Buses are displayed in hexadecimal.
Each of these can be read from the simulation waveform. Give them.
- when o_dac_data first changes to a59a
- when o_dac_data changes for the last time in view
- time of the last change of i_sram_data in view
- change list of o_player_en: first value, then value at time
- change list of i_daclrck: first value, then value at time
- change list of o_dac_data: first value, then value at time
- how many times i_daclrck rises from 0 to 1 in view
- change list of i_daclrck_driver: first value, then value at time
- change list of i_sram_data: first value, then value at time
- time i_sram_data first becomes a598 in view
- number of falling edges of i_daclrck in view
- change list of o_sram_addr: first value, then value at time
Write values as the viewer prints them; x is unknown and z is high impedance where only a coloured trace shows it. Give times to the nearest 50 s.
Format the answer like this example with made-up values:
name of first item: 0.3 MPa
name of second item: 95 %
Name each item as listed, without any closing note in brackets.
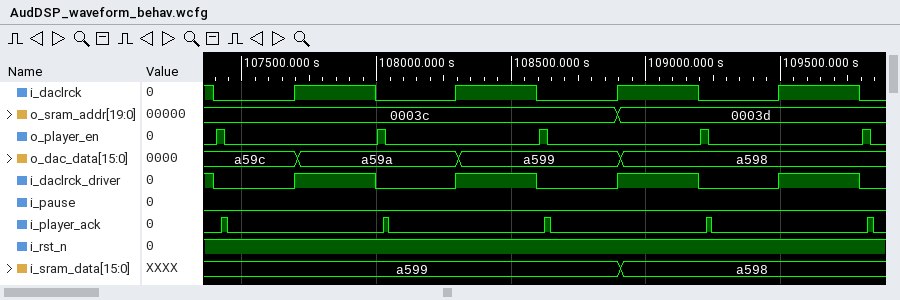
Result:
when o_dac_data first changes to a59a: 107700 s
when o_dac_data changes for the last time in view: 108900 s
time of the last change of i_sram_data in view: 108900 s
change list of o_player_en: first value, then value at time: 0, 1 at 107400 s, 0 at 107450 s, 1 at 108000 s, 0 at 108050 s, 1 at 108600 s, 0 at 108650 s, 1 at 109200 s, 0 at 109250 s, 1 at 109800 s, 0 at 109850 s
change list of i_daclrck: first value, then value at time: 1, 0 at 107400 s, 1 at 107700 s, 0 at 108000 s, 1 at 108300 s, 0 at 108600 s, 1 at 108900 s, 0 at 109200 s, 1 at 109500 s, 0 at 109800 s
change list of o_dac_data: first value, then value at time: a59c, a59a at 107700 s, a599 at 108300 s, a598 at 108900 s
how many times i_daclrck rises from 0 to 1 in view: 4
change list of i_daclrck_driver: first value, then value at time: 1, 0 at 107400 s, 1 at 107700 s, 0 at 108000 s, 1 at 108300 s, 0 at 108600 s, 1 at 108900 s, 0 at 109200 s, 1 at 109500 s, 0 at 109800 s
change list of i_sram_data: first value, then value at time: a599, a598 at 108900 s
time i_sram_data first becomes a598 in view: 108900 s
number of falling edges of i_daclrck in view: 5
change list of o_sram_addr: first value, then value at time: 0003c, 0003d at 108900 s
